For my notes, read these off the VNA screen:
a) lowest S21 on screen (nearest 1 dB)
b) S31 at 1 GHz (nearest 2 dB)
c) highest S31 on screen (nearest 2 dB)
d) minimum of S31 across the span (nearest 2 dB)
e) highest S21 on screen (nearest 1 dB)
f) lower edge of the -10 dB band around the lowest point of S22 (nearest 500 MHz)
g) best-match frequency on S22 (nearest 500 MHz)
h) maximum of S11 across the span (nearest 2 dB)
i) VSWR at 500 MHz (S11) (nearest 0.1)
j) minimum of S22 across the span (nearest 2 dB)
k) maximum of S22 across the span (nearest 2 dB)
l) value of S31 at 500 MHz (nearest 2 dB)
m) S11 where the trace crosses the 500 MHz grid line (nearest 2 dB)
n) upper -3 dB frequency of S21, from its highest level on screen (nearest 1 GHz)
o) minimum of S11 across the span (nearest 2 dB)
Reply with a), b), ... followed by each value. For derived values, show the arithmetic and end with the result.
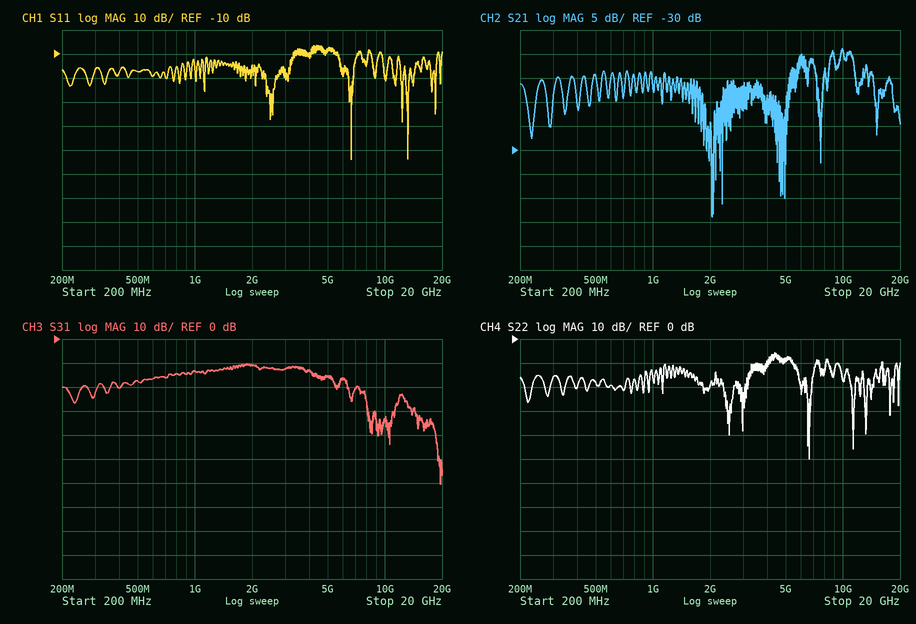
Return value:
a) -44 dB
b) -14 dB
c) -10 dB
d) -60 dB
e) -9 dB
f) 5.5 GHz
g) 6.5 GHz
h) -6 dB
i) |Γ| = 10^(-18/20) = 0.1259; VSWR = (1 + 0.1259)/(1 − 0.1259) ≈ 1.3
j) -50 dB
k) -6 dB
l) -18 dB
m) -18 dB
n) 11 GHz
o) -54 dB
